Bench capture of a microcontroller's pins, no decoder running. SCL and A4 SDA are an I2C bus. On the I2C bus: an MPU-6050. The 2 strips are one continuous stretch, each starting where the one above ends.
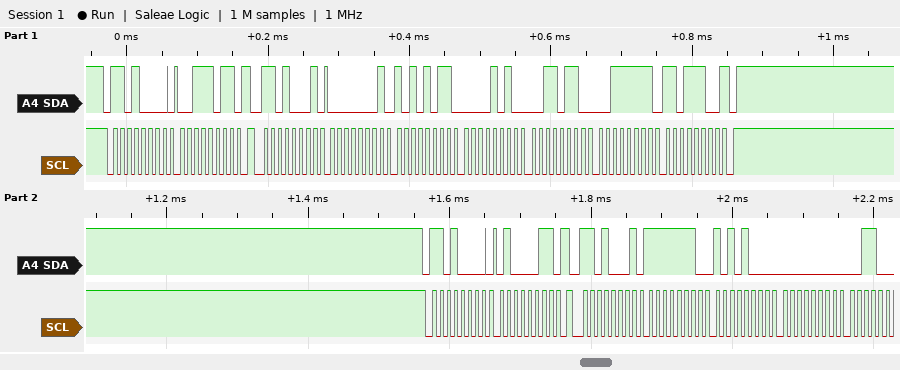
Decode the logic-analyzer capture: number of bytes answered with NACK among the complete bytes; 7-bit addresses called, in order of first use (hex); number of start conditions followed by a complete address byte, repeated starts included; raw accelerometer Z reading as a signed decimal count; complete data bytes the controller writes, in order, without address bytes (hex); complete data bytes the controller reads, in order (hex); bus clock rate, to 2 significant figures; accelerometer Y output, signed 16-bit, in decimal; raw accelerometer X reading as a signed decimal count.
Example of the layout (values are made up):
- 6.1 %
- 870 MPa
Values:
- 1
- 0x68
- 4
- 16348
- 3B 43
- 01 AB 0A 36 3F DC FE A8 00
- 100 kHz
- 2614
- 427
